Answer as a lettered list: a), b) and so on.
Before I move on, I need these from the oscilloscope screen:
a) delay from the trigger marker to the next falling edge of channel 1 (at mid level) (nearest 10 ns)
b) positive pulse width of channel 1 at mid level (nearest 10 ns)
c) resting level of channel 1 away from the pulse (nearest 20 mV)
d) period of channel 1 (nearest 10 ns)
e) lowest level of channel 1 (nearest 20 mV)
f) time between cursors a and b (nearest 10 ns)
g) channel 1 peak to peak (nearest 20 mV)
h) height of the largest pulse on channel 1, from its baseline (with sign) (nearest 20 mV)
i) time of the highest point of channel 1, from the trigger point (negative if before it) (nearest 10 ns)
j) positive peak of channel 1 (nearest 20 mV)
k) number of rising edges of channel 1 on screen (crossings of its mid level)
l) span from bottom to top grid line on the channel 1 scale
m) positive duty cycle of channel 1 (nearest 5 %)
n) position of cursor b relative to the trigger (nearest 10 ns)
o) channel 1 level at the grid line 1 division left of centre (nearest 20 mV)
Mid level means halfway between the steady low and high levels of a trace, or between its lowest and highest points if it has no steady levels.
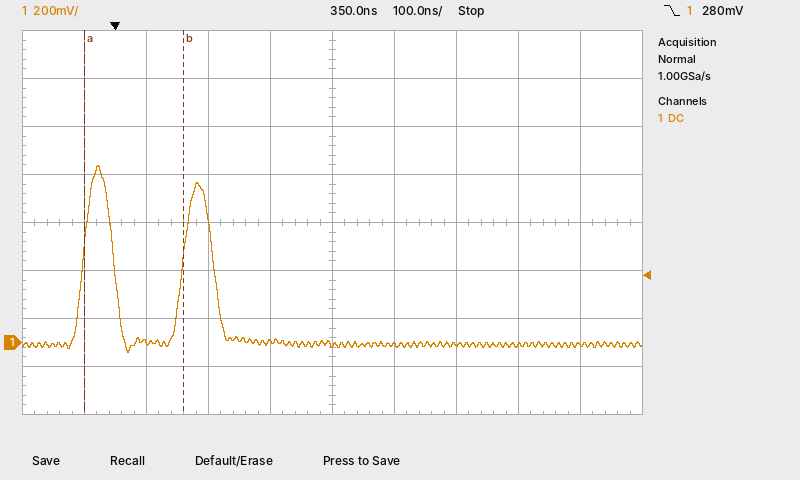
a) 160 ns
b) 50 ns
c) 0 mV
d) 160 ns
e) -40 mV
f) 160 ns
g) 780 mV
h) +740 mV
i) -30 ns
j) 740 mV
k) 2
l) 1.6 V
m) 30 %
n) +110 ns
o) 0 mV
